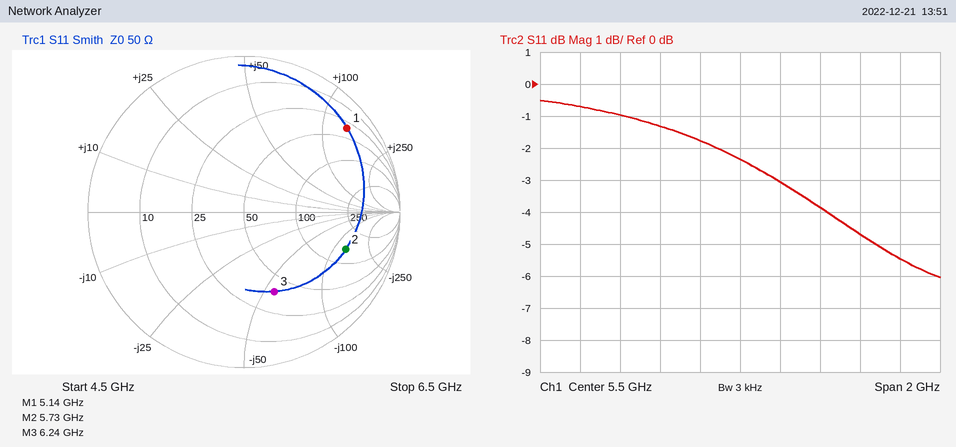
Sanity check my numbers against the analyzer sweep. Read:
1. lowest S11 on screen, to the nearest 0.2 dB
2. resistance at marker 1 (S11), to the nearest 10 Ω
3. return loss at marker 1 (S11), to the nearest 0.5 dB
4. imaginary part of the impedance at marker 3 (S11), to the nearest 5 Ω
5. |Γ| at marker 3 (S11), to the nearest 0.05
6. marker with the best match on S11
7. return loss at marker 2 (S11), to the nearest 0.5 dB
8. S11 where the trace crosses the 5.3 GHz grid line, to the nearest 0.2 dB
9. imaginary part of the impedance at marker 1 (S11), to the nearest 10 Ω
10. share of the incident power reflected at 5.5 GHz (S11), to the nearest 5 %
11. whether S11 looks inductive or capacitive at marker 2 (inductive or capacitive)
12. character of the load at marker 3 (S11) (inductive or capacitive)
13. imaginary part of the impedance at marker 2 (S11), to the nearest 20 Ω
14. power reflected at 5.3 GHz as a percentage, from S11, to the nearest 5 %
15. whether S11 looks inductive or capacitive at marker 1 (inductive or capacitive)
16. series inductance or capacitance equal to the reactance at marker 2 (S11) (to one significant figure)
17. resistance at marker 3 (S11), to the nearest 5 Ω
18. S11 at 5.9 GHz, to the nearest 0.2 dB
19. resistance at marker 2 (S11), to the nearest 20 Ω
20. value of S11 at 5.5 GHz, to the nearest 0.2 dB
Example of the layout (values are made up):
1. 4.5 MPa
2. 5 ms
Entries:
1. -6.0 dB
2. 30 Ω
3. 1.5 dB
4. -55 Ω
5. 0.55
6. marker 3
7. 3.0 dB
8. -1.8 dB
9. +130 Ω
10. 60 %
11. capacitive
12. capacitive
13. -140 Ω
14. 65 %
15. inductive
16. 200 fF
17. 40 Ω
18. -3.8 dB
19. 140 Ω
20. -2.4 dB
